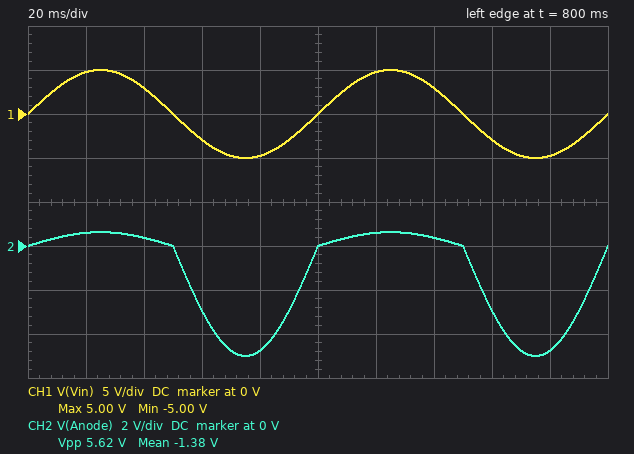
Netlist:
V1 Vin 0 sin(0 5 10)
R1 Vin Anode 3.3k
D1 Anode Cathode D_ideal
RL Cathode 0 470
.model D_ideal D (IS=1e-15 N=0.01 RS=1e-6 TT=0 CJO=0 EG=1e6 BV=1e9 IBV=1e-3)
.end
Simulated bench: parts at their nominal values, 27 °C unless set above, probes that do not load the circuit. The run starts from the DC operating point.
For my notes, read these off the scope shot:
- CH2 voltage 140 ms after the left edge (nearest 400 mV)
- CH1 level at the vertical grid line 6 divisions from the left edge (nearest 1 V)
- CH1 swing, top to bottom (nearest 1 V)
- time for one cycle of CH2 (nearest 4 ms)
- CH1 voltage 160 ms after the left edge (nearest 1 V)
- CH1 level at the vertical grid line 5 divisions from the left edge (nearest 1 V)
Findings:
400 mV
5 V
10 V
100 ms
-3 V
0 V
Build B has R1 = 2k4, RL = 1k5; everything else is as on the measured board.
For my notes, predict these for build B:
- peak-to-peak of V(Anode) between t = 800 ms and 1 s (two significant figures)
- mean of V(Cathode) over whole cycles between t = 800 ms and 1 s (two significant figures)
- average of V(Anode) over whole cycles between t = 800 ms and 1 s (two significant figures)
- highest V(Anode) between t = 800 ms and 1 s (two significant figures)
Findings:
6.9 V
610 mV
-980 mV
1.9 V
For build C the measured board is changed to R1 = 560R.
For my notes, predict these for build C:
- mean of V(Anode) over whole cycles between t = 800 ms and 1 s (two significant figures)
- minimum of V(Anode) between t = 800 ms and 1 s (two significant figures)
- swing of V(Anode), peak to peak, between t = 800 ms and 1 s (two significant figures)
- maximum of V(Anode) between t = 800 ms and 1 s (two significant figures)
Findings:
-860 mV
-5.0 V
7.3 V
2.3 V
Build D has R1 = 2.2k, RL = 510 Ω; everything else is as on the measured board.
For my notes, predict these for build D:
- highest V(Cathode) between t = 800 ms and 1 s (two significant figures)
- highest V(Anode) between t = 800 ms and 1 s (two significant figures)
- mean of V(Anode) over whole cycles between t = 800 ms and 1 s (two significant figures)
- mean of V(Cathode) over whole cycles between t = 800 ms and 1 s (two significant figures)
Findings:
940 mV
950 mV
-1.3 V
300 mV
